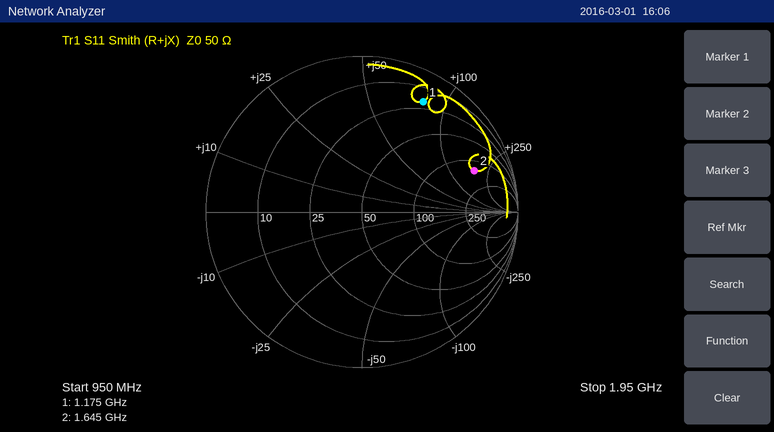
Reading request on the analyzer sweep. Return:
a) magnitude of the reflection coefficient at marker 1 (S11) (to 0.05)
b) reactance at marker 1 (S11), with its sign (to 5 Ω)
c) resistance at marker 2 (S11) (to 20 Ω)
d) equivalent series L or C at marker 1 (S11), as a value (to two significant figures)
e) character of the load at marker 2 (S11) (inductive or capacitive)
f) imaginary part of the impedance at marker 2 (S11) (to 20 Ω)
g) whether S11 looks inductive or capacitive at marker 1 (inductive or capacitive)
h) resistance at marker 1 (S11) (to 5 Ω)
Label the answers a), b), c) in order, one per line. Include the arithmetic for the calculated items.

a) 0.80
b) +80 Ω
c) 140 Ω
d) L = 80 Ω/(2π × 1.175 GHz) ≈ 11 nH
e) inductive
f) +180 Ω
g) inductive
h) 20 Ω
